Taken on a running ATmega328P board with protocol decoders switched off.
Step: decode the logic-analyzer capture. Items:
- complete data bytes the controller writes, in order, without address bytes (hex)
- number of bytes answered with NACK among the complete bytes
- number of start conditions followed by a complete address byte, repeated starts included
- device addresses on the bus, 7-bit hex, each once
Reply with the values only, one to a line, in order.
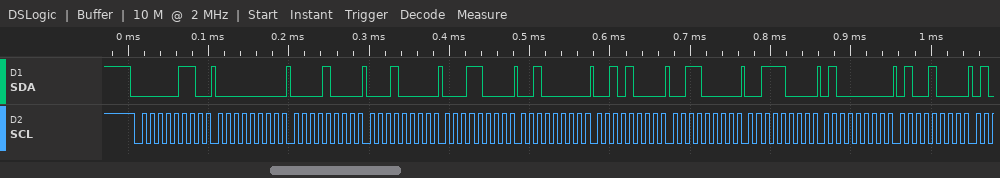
00 08 10 18 20 28 30 38 40 48
0
1
0x03
